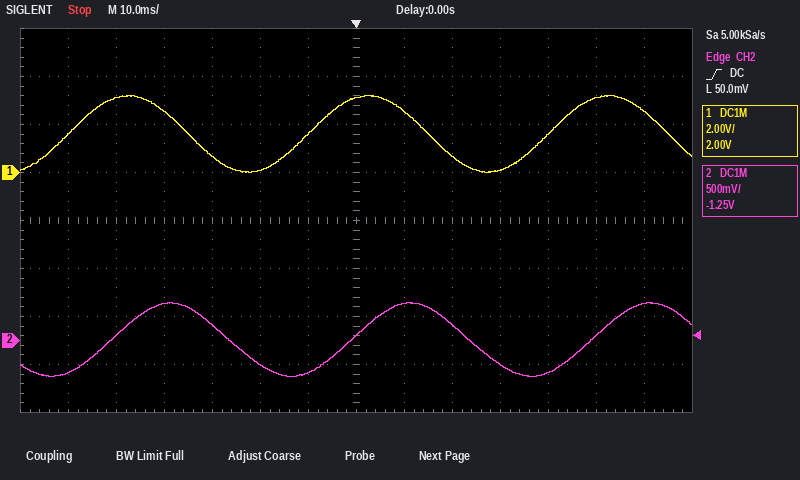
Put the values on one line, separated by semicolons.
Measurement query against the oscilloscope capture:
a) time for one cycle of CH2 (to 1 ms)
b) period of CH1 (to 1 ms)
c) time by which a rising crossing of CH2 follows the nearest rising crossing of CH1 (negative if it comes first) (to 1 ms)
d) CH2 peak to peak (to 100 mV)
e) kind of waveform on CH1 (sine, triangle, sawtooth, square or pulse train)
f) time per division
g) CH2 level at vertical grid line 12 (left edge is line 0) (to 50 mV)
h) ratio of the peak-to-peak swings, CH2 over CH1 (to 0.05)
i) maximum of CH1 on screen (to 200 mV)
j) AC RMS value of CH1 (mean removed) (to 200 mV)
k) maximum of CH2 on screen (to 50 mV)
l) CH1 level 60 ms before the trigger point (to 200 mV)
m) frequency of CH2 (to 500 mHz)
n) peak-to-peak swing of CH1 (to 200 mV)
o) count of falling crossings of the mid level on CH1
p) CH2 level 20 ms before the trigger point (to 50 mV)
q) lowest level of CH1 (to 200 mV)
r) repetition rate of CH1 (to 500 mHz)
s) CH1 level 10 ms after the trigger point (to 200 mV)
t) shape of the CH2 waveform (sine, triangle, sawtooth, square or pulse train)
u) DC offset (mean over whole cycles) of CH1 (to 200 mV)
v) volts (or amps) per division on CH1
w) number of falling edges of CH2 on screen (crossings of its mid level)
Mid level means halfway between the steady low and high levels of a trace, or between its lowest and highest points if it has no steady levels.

50 ms; 50 ms; +9 ms; 800 mV; sine; 10 ms; 50 mV; 0.25; 3.2 V; 1.2 V; 400 mV; 1.6 V; 20.0 Hz; 3.2 V; 3; -250 mV; 0.0 V; 20.0 Hz; 2.6 V; sine; 1.6 V; 2 V; 2
